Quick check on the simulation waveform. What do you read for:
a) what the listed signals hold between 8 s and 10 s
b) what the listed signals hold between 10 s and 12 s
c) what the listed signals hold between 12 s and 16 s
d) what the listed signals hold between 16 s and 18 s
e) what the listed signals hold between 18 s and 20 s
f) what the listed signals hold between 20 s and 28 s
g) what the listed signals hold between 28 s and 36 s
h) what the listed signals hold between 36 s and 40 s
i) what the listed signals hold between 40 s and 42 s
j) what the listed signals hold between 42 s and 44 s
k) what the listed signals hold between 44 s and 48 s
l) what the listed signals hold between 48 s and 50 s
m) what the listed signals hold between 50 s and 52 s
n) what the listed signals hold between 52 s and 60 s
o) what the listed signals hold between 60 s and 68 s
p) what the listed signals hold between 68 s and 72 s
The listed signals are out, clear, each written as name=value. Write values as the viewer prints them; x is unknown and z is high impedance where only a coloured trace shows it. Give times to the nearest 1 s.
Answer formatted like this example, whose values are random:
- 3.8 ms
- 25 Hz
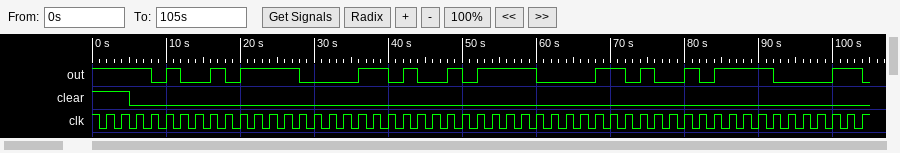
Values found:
- out=0, clear=0
- out=1, clear=0
- out=0, clear=0
- out=1, clear=0
- out=0, clear=0
- out=1, clear=0
- out=0, clear=0
- out=1, clear=0
- out=0, clear=0
- out=1, clear=0
- out=0, clear=0
- out=1, clear=0
- out=0, clear=0
- out=1, clear=0
- out=0, clear=0
- out=1, clear=0
